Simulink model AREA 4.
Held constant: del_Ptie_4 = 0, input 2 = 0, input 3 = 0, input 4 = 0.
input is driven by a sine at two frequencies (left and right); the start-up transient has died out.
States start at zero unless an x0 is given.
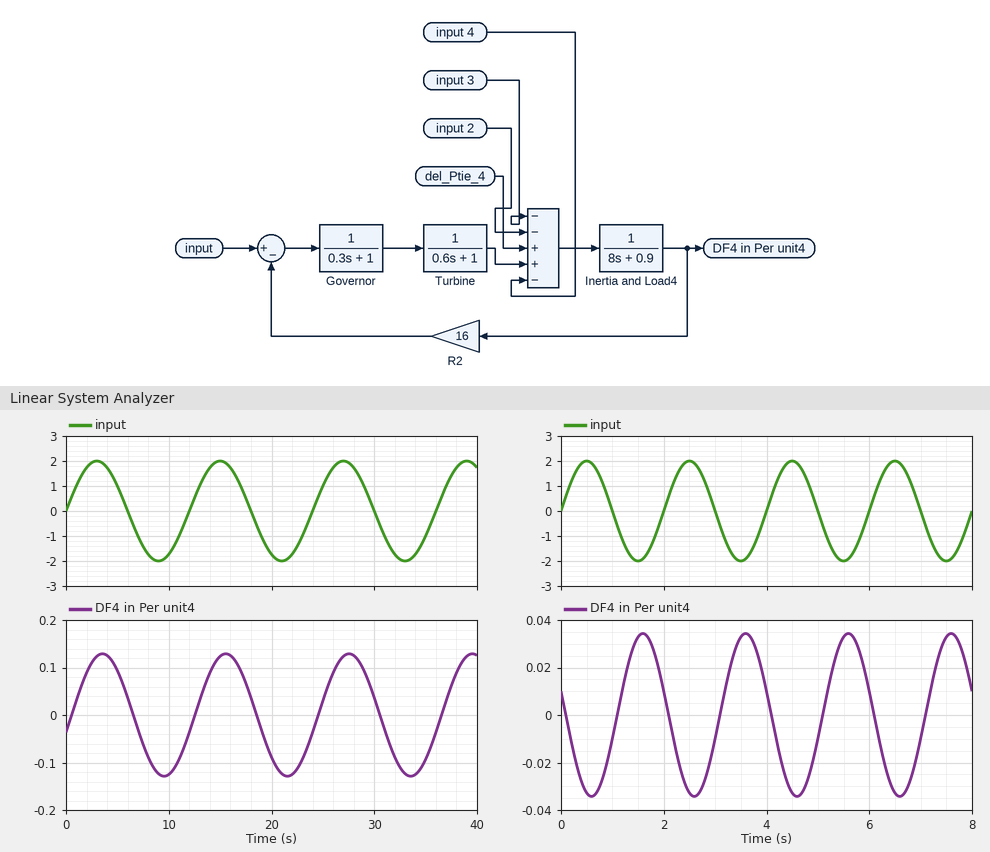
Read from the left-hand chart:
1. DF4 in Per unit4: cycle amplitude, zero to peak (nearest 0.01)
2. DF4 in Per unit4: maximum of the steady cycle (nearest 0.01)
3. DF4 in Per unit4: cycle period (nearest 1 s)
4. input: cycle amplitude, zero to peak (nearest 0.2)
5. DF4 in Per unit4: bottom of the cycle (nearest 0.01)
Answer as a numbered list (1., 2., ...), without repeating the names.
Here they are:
1. 0.13
2. 0.13
3. 12 s
4. 2.0
5. -0.13
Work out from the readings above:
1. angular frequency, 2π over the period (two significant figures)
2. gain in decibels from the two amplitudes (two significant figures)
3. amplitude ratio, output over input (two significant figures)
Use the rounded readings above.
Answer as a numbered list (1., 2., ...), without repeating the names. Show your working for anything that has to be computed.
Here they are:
1. 2π / 12 = 0.52 rad/s
2. 20 log10(0.13 / 2) = -24 dB
3. 0.13 / 2 = 0.065
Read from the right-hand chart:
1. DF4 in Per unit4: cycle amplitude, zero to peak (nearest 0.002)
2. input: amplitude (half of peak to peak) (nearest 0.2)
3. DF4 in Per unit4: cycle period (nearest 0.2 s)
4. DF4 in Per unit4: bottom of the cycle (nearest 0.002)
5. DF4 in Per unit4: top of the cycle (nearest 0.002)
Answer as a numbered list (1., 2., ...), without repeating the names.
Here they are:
1. 0.034
2. 2.0
3. 2.0 s
4. -0.034
5. 0.034
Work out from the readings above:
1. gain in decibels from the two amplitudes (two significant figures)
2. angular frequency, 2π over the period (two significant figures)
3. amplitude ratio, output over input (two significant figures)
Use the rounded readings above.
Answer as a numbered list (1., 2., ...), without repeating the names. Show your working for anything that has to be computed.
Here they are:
1. 20 log10(0.034 / 2) = -35 dB
2. 2π / 2 = 3.1 rad/s
3. 0.034 / 2 = 0.017
